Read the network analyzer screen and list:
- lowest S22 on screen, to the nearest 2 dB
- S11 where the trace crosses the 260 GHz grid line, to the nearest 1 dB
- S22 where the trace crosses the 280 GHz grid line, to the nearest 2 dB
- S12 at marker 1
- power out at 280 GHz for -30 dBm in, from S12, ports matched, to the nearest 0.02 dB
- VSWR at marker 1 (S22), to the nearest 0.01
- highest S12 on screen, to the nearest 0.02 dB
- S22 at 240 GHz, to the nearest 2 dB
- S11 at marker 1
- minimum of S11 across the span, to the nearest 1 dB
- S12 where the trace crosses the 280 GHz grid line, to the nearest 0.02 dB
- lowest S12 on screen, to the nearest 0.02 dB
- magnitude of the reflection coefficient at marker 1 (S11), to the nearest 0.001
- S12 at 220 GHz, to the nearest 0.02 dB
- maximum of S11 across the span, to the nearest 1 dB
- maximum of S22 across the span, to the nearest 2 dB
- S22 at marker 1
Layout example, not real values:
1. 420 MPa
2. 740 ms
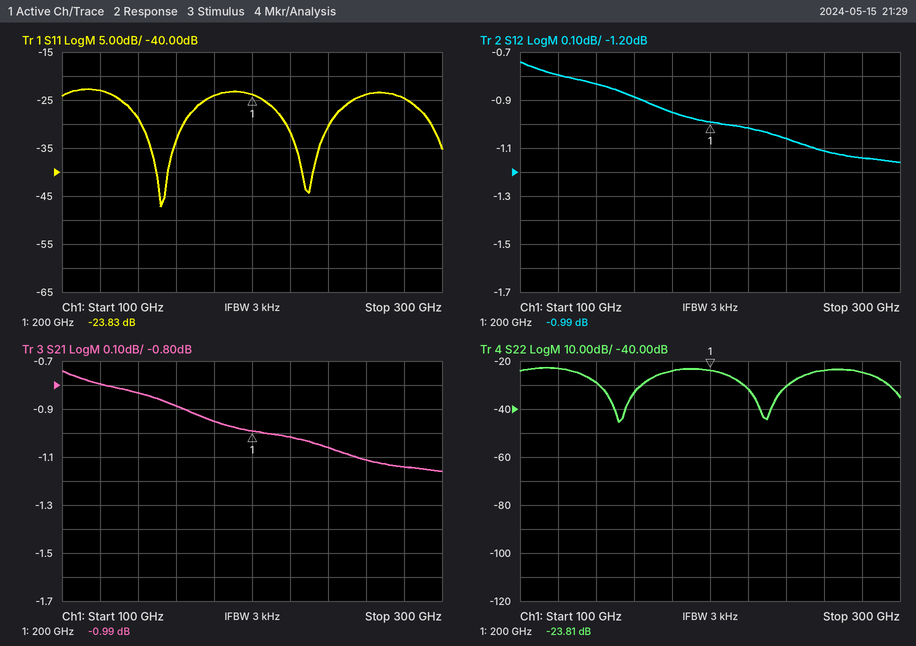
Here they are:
1. -46 dB
2. -24 dB
3. -24 dB
4. -0.99 dB
5. -31.14 dBm
6. 1.14
7. -0.74 dB
8. -30 dB
9. -23.83 dB
10. -47 dB
11. -1.14 dB
12. -1.16 dB
13. 0.064
14. -1.02 dB
15. -23 dB
16. -22 dB
17. -23.81 dB
